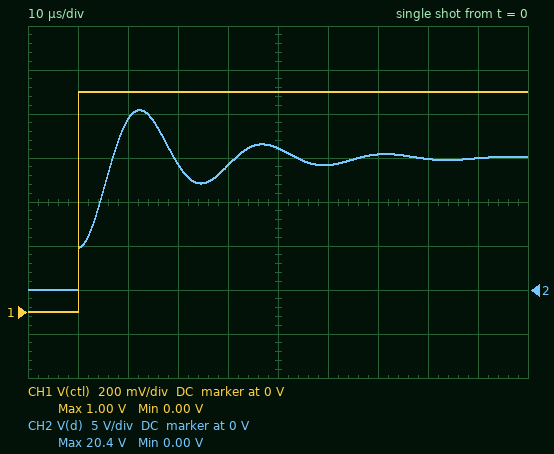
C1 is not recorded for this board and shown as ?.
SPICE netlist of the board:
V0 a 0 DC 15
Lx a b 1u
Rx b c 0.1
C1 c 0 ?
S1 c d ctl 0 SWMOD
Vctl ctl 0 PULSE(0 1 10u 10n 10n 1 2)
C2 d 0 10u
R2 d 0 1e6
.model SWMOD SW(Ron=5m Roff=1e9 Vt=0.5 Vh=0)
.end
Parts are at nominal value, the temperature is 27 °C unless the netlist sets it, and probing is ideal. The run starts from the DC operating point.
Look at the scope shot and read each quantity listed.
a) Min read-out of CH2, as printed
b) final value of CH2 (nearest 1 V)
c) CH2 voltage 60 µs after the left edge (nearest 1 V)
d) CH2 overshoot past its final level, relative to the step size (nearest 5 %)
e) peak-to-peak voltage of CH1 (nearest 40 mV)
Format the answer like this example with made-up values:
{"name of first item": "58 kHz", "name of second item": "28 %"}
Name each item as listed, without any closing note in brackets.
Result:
{"Min read-out of CH2, as printed": "0.00 V", "final value of CH2": "15 V", "CH2 voltage 60 µs after the left edge": "14 V", "CH2 overshoot past its final level, relative to the step size": "35 %", "peak-to-peak voltage of CH1": "1.00 V"}
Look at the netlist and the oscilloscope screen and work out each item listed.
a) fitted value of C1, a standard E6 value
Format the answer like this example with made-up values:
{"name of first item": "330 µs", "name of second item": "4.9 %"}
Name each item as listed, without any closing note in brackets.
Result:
{"fitted value of C1, a standard E6 value": "4.7 µF"}
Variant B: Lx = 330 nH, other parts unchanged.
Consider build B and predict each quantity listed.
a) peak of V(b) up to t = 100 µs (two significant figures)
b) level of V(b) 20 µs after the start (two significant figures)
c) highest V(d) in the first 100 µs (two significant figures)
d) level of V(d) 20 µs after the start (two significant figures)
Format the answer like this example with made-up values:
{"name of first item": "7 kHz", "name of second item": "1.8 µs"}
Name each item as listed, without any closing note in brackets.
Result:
{"peak of V(b) up to t = 100 µs": "19 V", "level of V(b) 20 µs after the start": "15 V", "highest V(d) in the first 100 µs": "18 V", "level of V(d) 20 µs after the start": "17 V"}
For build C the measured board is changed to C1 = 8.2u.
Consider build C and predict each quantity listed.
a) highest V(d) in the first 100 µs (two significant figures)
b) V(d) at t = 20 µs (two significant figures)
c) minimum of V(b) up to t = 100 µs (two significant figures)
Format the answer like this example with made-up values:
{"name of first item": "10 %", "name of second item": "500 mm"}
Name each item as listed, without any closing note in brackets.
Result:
{"highest V(d) in the first 100 µs": "19 V", "V(d) at t = 20 µs": "17 V", "minimum of V(b) up to t = 100 µs": "6.9 V"}
